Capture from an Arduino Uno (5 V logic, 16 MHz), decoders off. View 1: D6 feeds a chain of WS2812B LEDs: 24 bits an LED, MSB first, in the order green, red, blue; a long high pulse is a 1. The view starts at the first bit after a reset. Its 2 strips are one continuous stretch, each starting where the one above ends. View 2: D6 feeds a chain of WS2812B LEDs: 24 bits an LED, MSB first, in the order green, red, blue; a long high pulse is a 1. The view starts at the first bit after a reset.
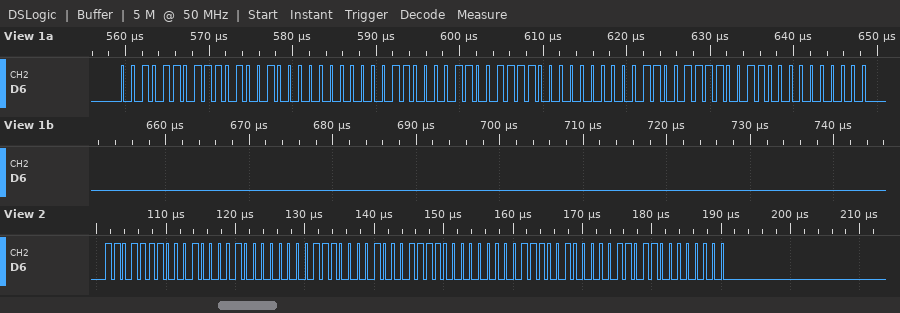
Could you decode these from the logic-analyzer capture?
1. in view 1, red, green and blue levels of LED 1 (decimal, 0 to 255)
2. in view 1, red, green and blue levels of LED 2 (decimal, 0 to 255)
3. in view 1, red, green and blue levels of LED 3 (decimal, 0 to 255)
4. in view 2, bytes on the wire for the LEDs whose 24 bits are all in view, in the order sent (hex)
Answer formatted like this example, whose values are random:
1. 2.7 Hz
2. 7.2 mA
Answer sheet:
1. 210, 45, 0
2. 207, 48, 0
3. 204, 51, 0
4. DE 21 00 E1 1E 00 E4 1B 00
